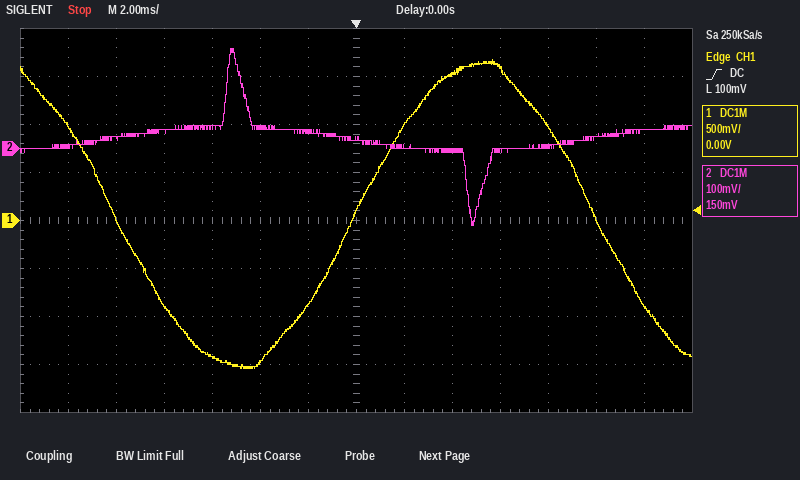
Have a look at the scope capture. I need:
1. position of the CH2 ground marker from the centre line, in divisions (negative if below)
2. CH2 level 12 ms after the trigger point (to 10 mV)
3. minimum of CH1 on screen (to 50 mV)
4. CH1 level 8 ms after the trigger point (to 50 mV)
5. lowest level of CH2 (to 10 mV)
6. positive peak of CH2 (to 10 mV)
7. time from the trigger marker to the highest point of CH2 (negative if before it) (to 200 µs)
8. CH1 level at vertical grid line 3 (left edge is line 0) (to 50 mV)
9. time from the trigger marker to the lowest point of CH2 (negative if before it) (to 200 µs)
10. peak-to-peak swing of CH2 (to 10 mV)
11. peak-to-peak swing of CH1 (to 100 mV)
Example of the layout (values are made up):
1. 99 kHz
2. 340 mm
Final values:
1. +1.5 div
2. 40 mV
3. -1.55 V
4. 1.00 V
5. -160 mV
6. 210 mV
7. -5.2 ms
8. -900 mV
9. +4.8 ms
10. 370 mV
11. 3.20 V
